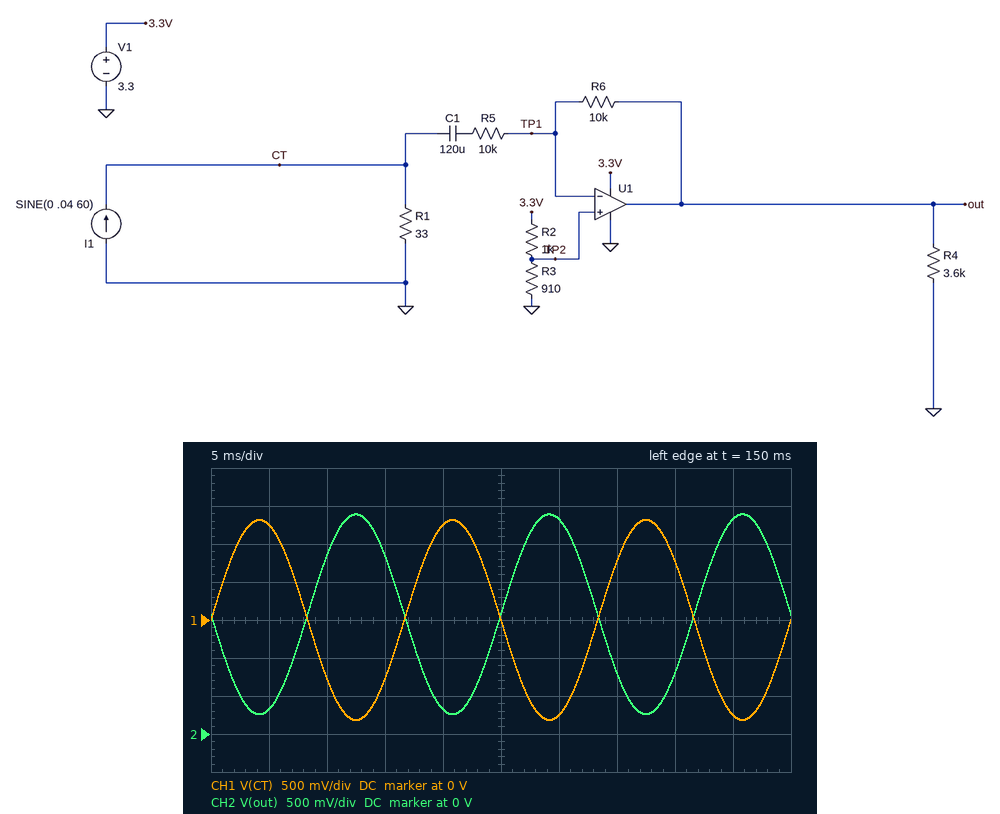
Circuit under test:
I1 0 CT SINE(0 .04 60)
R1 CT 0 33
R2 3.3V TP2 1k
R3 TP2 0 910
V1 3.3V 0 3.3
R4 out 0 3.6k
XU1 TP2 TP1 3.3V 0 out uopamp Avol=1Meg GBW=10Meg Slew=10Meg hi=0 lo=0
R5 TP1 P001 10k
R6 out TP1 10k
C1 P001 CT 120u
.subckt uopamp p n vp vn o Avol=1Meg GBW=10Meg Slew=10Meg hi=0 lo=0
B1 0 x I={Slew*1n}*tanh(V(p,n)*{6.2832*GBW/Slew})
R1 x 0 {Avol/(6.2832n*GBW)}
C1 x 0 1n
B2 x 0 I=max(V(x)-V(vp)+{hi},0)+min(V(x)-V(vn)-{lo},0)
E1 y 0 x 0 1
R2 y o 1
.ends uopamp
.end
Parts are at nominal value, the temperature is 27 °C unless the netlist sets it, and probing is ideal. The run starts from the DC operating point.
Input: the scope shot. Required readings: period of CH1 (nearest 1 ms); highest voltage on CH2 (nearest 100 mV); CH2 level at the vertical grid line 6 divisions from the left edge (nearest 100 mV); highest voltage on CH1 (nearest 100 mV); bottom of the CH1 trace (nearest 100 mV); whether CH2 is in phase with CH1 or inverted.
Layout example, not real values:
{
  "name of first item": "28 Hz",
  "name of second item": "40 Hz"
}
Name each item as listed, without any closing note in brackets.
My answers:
{
  "period of CH1": "17 ms",
  "highest voltage on CH2": "2.9 V",
  "CH2 level at the vertical grid line 6 divisions from the left edge": "2.8 V",
  "highest voltage on CH1": "1.3 V",
  "bottom of the CH1 trace": "-1.3 V",
  "whether CH2 is in phase with CH1 or inverted": "inverted"
}
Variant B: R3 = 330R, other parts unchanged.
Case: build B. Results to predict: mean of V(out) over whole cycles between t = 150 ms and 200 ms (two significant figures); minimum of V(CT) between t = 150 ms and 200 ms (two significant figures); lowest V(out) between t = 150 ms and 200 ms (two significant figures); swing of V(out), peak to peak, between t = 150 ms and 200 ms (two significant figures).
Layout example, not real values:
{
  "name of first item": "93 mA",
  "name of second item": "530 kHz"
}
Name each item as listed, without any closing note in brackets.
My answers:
{
  "mean of V(out) over whole cycles between t = 150 ms and 200 ms": "910 mV",
  "minimum of V(CT) between t = 150 ms and 200 ms": "-1.3 V",
  "lowest V(out) between t = 150 ms and 200 ms": "-9.0 mV",
  "swing of V(out), peak to peak, between t = 150 ms and 200 ms": "2.1 V"
}
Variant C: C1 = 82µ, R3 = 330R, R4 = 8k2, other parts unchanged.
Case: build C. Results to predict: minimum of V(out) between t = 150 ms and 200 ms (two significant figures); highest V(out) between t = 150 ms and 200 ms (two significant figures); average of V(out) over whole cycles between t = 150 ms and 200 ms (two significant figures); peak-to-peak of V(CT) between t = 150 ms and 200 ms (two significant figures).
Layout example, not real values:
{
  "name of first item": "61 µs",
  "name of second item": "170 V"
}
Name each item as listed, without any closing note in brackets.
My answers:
{
  "minimum of V(out) between t = 150 ms and 200 ms": "-9.0 mV",
  "highest V(out) between t = 150 ms and 200 ms": "2.1 V",
  "average of V(out) over whole cycles between t = 150 ms and 200 ms": "910 mV",
  "peak-to-peak of V(CT) between t = 150 ms and 200 ms": "2.6 V"
}
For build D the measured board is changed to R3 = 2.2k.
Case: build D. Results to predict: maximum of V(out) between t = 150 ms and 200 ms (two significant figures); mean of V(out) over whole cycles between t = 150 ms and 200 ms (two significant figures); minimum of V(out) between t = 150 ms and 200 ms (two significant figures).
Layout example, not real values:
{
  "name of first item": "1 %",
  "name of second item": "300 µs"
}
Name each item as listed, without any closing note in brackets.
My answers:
{
  "maximum of V(out) between t = 150 ms and 200 ms": "3.3 V",
  "mean of V(out) over whole cycles between t = 150 ms and 200 ms": "2.2 V",
  "minimum of V(out) between t = 150 ms and 200 ms": "960 mV"
}
